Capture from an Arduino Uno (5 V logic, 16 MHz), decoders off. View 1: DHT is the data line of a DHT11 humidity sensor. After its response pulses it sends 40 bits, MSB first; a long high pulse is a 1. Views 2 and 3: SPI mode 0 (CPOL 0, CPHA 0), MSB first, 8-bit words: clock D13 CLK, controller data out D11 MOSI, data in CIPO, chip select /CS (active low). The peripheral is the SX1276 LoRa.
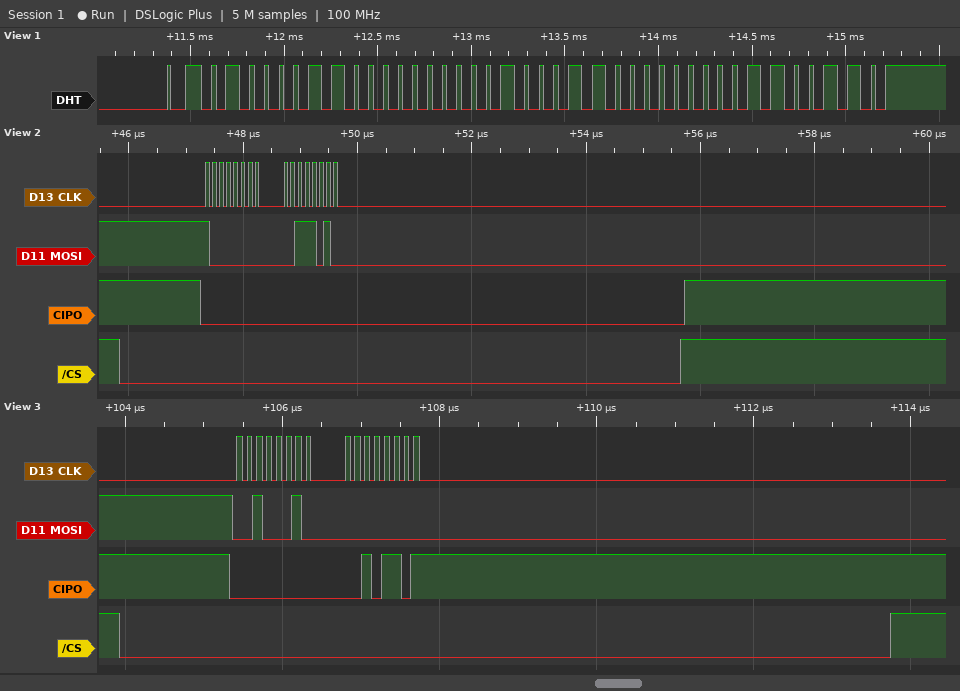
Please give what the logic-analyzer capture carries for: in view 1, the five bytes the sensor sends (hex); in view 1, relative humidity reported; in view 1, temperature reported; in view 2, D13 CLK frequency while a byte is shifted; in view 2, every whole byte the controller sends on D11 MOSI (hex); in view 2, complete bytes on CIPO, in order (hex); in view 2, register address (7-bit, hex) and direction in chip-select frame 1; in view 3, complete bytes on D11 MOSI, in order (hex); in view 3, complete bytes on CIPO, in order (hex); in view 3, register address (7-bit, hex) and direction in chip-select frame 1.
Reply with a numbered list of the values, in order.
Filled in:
1. 43 00 23 00 66
2. 67 %
3. 35.0 °C
4. 8 MHz
5. 0x80 0x3A
6. 0x00 0x00
7. 0x00 write
8. 22 00
9. 00 2D
10. 0x22 read
